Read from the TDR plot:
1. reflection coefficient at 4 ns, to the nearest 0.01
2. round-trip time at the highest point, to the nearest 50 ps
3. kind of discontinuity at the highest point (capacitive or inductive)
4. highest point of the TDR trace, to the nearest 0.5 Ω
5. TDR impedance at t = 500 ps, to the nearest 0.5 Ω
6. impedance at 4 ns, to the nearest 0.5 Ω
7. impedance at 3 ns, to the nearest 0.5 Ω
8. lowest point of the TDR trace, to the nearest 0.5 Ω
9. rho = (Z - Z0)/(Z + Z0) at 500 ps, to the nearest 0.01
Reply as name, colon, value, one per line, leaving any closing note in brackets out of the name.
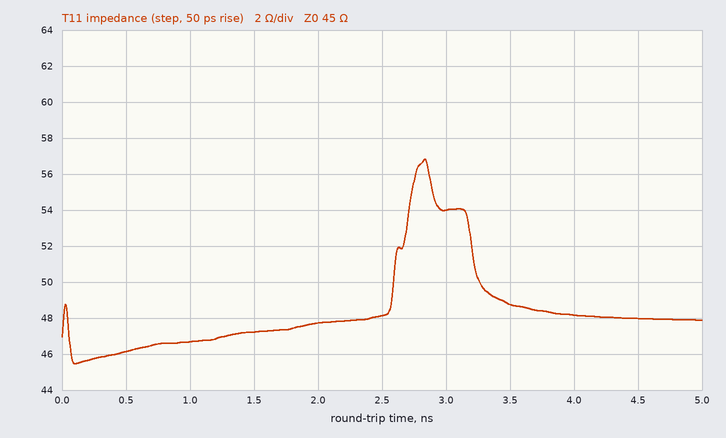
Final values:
reflection coefficient at 4 ns, to the nearest 0.01: +0.03
round-trip time at the highest point, to the nearest 50 ps: 2.85 ns
kind of discontinuity at the highest point: inductive
highest point of the TDR trace, to the nearest 0.5 Ω: 57.0 Ω
TDR impedance at t = 500 ps, to the nearest 0.5 Ω: 46.0 Ω
impedance at 4 ns, to the nearest 0.5 Ω: 48.0 Ω
impedance at 3 ns, to the nearest 0.5 Ω: 54.0 Ω
lowest point of the TDR trace, to the nearest 0.5 Ω: 45.5 Ω
rho = (Z - Z0)/(Z + Z0) at 500 ps, to the nearest 0.01: +0.01
